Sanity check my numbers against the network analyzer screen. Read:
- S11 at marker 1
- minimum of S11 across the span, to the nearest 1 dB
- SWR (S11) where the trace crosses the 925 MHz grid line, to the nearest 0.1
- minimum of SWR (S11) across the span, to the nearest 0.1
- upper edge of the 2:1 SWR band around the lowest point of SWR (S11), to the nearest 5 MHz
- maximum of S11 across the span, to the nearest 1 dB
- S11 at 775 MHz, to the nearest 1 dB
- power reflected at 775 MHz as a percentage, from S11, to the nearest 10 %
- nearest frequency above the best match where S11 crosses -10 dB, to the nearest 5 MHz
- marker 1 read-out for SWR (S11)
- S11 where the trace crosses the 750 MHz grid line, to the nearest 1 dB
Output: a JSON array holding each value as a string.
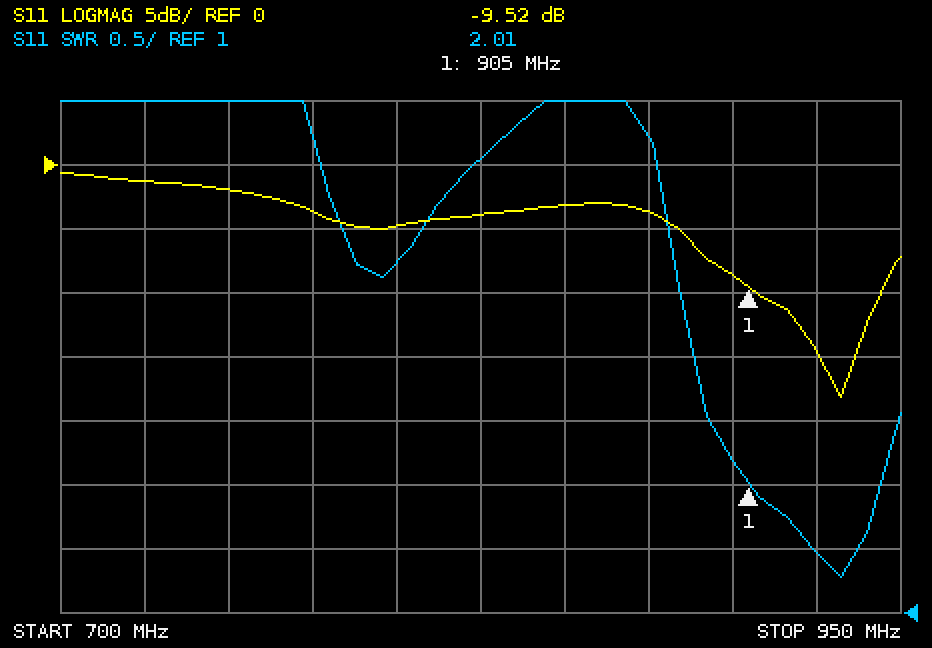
["-9.52 dB", "-18 dB", "1.5", "1.3", "945 MHz", "-1 dB", "-4 dB", "40 %", "945 MHz", "2.01", "-2 dB"]
